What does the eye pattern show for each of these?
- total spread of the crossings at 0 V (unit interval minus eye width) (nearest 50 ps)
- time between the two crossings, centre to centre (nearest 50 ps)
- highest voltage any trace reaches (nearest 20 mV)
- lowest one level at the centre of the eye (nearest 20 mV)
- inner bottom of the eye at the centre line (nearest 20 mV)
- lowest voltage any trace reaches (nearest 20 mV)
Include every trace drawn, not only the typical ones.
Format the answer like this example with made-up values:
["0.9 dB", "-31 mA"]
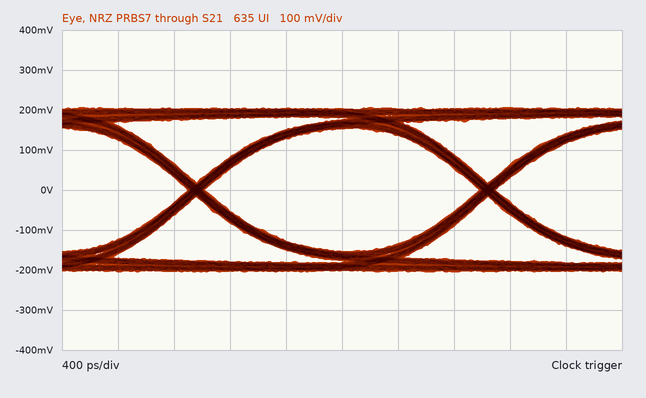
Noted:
["100 ps", "2.10 ns", "200 mV", "160 mV", "-160 mV", "-200 mV"]
